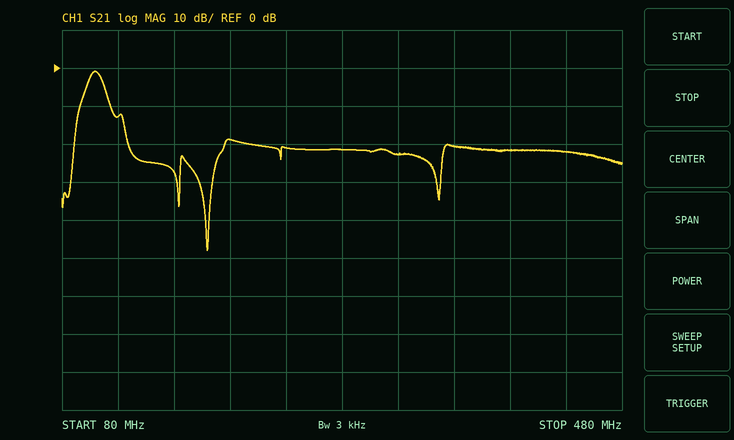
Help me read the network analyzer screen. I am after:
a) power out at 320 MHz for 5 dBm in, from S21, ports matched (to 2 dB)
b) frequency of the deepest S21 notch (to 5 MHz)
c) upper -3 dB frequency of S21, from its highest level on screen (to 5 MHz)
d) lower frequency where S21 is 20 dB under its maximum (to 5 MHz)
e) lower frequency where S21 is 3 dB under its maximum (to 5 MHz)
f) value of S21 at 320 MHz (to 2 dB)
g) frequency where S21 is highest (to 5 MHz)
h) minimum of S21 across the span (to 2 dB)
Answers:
-18 dBm
185 MHz
110 MHz
90 MHz
100 MHz
-22 dB
105 MHz
-48 dB
